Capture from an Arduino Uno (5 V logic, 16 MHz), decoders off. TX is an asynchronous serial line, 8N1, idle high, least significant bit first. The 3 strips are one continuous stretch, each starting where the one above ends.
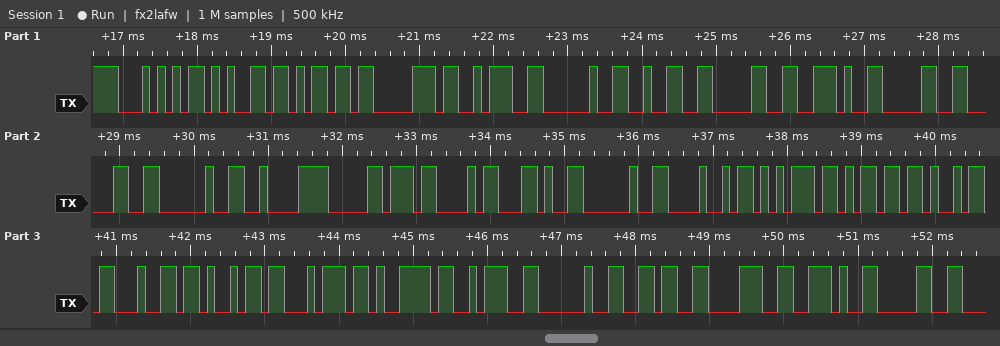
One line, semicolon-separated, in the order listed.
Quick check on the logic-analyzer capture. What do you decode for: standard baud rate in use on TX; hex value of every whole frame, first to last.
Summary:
9600 baud; 54 65 6D 70 3A 20 32 30 2E 30 30 20 C2 B0 43 2C 20 48 75 6D 69 64 69 74 79 3A 20 36 38 2E 30
